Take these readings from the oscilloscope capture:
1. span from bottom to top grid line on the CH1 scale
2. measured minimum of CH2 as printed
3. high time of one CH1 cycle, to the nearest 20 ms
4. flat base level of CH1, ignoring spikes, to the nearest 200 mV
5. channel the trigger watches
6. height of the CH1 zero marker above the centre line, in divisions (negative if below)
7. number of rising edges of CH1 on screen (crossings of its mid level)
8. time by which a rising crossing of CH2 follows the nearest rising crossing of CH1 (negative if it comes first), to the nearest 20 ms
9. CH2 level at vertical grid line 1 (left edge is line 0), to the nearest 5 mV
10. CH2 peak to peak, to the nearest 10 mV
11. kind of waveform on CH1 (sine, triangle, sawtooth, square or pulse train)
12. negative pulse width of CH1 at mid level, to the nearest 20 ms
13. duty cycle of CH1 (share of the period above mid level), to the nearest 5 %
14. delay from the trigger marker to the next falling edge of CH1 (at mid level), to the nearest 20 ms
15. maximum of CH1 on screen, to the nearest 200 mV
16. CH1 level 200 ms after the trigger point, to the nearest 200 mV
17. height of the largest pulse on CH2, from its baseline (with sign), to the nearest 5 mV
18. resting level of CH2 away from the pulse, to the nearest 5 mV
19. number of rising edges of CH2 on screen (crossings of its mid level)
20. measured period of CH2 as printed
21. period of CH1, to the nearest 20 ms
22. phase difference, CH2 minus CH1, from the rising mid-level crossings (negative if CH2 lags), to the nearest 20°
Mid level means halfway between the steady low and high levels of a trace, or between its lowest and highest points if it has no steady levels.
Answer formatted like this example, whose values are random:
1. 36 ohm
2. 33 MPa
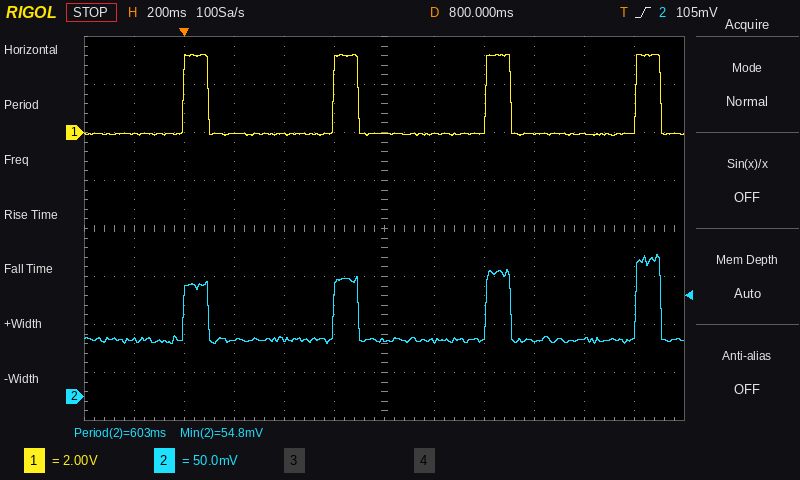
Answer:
1. 16 V
2. 54.8 mV
3. 100 ms
4. 0.0 V
5. CH2
6. +2.0 div
7. 4
8. 0 ms
9. 60 mV
10. 90 mV
11. pulse train
12. 500 ms
13. 15 %
14. 100 ms
15. 3.2 V
16. 0.0 V
17. +90 mV
18. 60 mV
19. 4
20. 603 ms
21. 600 ms
22. 0°
